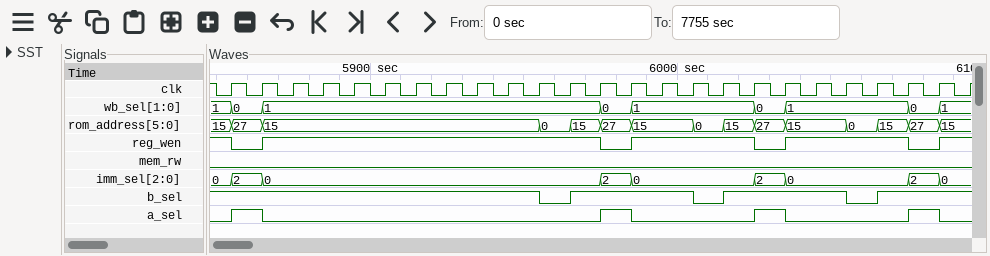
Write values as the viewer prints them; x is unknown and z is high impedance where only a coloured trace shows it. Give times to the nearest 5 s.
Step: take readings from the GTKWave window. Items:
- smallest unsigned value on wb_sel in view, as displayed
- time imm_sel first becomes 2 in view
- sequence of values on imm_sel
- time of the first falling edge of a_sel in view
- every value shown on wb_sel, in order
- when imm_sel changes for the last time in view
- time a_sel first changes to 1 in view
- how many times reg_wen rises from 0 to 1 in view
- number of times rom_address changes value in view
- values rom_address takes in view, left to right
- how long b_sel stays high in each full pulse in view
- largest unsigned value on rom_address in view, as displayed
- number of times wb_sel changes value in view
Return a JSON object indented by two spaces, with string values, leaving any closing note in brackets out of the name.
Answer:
{
  "smallest unsigned value on wb_sel in view, as displayed": "0",
  "time imm_sel first becomes 2 in view": "5855 s",
  "sequence of values on imm_sel": "0, 2, 0, 2, 0, 2, 0, 2, 0",
  "time of the first falling edge of a_sel in view": "5865 s",
  "every value shown on wb_sel, in order": "1, 0, 1, 0, 1, 0, 1, 0, 1",
  "when imm_sel changes for the last time in view": "6085 s",
  "time a_sel first changes to 1 in view": "5855 s",
  "how many times reg_wen rises from 0 to 1 in view": "4",
  "number of times rom_address changes value in view": "14",
  "values rom_address takes in view, left to right": "15, 27, 15, 0, 15, 27, 15, 0, 15, 27, 15, 0, 15, 27, 15",
  "how long b_sel stays high in each full pulse in view": "40 s, 40 s",
  "largest unsigned value on rom_address in view, as displayed": "27",
  "number of times wb_sel changes value in view": "8"
}
